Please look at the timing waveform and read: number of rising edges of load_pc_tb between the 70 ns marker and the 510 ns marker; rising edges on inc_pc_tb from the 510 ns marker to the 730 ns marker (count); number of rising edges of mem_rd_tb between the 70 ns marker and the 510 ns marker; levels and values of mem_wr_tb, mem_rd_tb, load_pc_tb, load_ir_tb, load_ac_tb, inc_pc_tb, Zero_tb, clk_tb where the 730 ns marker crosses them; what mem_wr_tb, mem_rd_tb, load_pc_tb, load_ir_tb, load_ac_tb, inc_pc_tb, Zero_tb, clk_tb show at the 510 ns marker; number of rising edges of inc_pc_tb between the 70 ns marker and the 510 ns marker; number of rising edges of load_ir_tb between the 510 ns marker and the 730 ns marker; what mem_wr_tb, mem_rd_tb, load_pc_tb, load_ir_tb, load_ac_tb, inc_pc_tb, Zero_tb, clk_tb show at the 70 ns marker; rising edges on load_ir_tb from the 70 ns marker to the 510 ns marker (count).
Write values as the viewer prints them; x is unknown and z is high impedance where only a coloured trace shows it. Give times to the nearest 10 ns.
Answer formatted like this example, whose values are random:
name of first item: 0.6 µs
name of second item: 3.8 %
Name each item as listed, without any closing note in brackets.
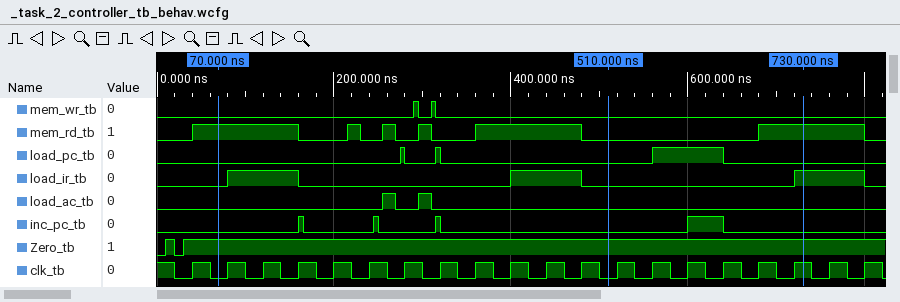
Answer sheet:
number of rising edges of load_pc_tb between the 70 ns marker and the 510 ns marker: 2
rising edges on inc_pc_tb from the 510 ns marker to the 730 ns marker: 1
number of rising edges of mem_rd_tb between the 70 ns marker and the 510 ns marker: 4
levels and values of mem_wr_tb, mem_rd_tb, load_pc_tb, load_ir_tb, load_ac_tb, inc_pc_tb, Zero_tb, clk_tb where the 730 ns marker crosses them: mem_wr_tb=0, mem_rd_tb=1, load_pc_tb=0, load_ir_tb=1, load_ac_tb=0, inc_pc_tb=0, Zero_tb=1, clk_tb=1
what mem_wr_tb, mem_rd_tb, load_pc_tb, load_ir_tb, load_ac_tb, inc_pc_tb, Zero_tb, clk_tb show at the 510 ns marker: mem_wr_tb=0, mem_rd_tb=0, load_pc_tb=0, load_ir_tb=0, load_ac_tb=0, inc_pc_tb=0, Zero_tb=1, clk_tb=0
number of rising edges of inc_pc_tb between the 70 ns marker and the 510 ns marker: 3
number of rising edges of load_ir_tb between the 510 ns marker and the 730 ns marker: 1
what mem_wr_tb, mem_rd_tb, load_pc_tb, load_ir_tb, load_ac_tb, inc_pc_tb, Zero_tb, clk_tb show at the 70 ns marker: mem_wr_tb=0, mem_rd_tb=1, load_pc_tb=0, load_ir_tb=0, load_ac_tb=0, inc_pc_tb=0, Zero_tb=1, clk_tb=0
rising edges on load_ir_tb from the 70 ns marker to the 510 ns marker: 2
